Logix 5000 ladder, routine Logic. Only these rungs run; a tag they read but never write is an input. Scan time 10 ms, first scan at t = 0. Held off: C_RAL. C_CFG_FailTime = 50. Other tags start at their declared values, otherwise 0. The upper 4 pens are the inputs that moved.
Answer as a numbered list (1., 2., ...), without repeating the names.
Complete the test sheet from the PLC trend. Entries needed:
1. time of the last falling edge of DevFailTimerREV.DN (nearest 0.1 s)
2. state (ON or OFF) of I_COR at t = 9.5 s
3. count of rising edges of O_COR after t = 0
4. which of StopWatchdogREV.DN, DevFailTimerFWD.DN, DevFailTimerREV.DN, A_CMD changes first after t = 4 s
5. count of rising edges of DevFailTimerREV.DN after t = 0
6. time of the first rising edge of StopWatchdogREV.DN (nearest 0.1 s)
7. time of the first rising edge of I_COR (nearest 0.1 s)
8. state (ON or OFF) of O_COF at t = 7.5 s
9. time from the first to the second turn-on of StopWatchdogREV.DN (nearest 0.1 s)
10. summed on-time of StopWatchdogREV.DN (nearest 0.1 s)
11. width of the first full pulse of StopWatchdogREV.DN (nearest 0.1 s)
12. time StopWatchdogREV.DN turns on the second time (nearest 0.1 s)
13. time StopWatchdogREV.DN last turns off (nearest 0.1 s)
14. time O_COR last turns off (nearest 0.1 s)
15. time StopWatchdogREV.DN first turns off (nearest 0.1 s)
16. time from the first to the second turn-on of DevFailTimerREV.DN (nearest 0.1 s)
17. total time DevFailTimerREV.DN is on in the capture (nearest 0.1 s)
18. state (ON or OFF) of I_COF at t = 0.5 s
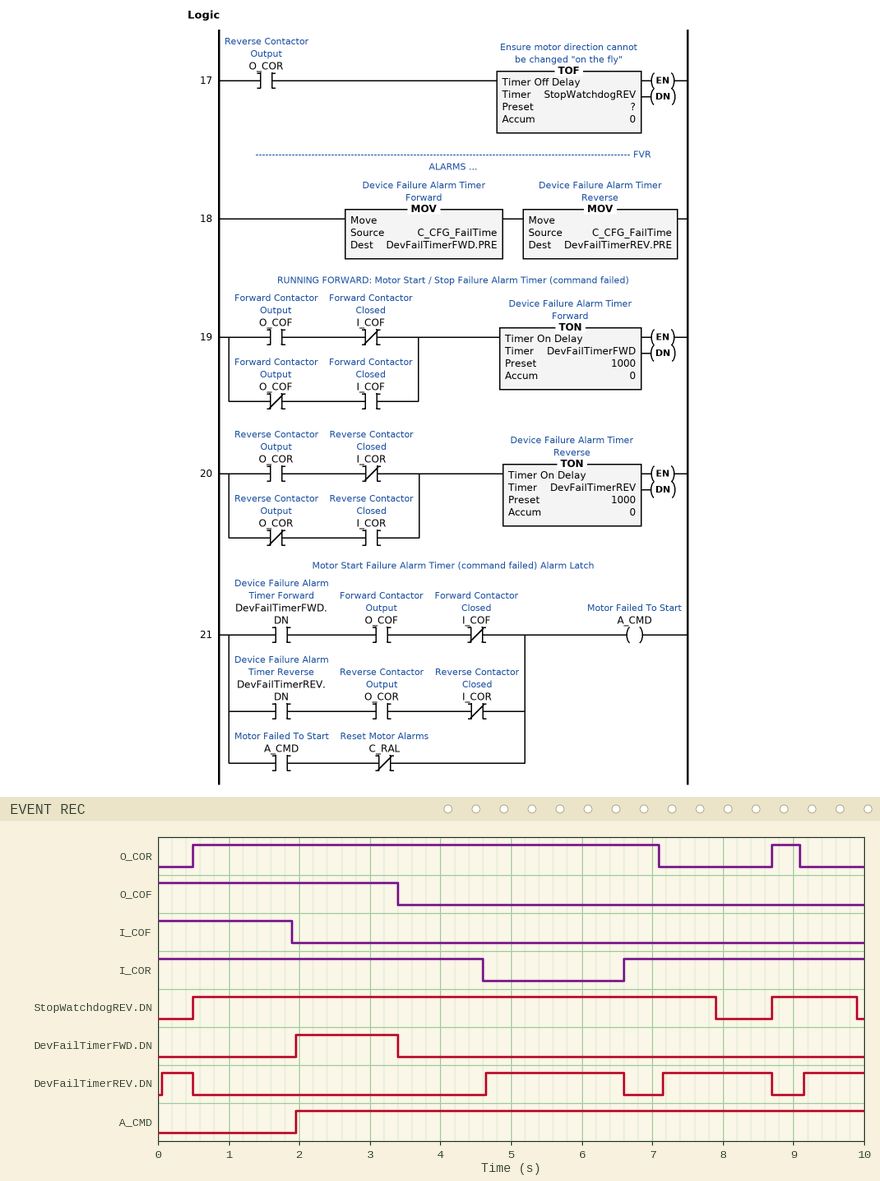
1. 8.7 s
2. ON
3. 2
4. DevFailTimerREV.DN
5. 4
6. 0.5 s
7. 6.6 s
8. OFF
9. 8.2 s
10. 8.6 s
11. 7.4 s
12. 8.7 s
13. 9.9 s
14. 9.1 s
15. 7.9 s
16. 4.6 s
17. 4.8 s
18. ON
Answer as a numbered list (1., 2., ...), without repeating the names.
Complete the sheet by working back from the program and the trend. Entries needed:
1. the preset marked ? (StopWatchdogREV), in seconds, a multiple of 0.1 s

1. 0.8 s
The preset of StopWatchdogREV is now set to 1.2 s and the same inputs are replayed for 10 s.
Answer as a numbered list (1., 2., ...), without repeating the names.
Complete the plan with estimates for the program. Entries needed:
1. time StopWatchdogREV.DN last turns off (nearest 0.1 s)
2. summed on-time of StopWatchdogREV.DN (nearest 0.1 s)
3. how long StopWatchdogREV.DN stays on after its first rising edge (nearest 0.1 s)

1. 8.3 s
2. 9.1 s
3. 7.8 s
